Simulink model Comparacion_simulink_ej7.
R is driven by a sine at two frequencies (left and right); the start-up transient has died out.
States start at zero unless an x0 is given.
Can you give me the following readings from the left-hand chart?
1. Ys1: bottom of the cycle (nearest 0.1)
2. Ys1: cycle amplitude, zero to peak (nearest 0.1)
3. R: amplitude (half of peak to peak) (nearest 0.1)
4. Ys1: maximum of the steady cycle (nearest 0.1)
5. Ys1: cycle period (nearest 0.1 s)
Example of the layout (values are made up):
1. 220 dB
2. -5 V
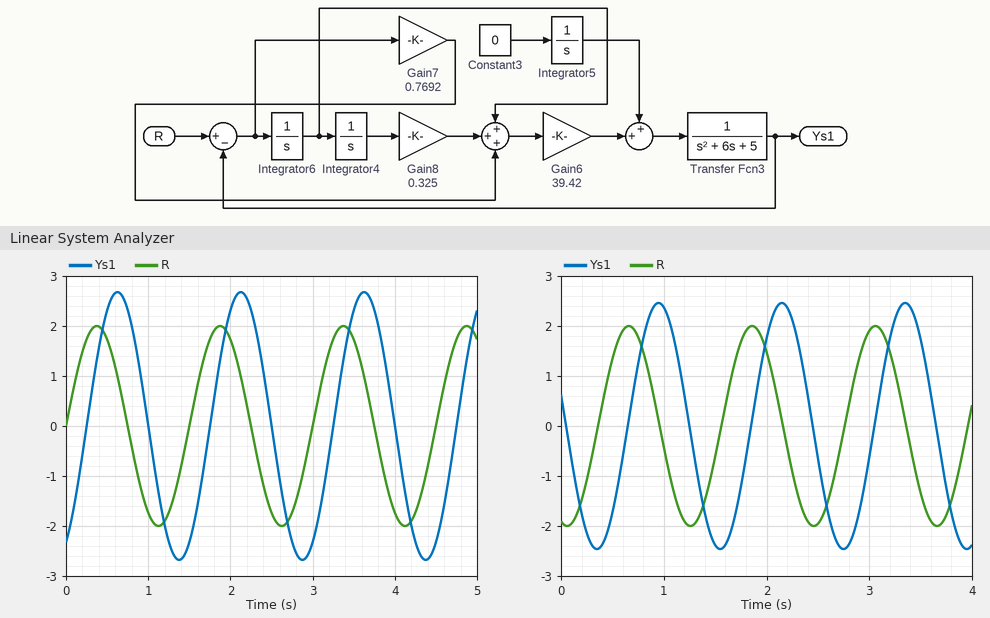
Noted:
1. -2.7
2. 2.7
3. 2.0
4. 2.7
5. 1.5 s
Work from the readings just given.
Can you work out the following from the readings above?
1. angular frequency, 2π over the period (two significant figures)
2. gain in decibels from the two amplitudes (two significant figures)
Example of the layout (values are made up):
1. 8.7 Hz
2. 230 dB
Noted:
1. 4.2 rad/s
2. 2.6 dB
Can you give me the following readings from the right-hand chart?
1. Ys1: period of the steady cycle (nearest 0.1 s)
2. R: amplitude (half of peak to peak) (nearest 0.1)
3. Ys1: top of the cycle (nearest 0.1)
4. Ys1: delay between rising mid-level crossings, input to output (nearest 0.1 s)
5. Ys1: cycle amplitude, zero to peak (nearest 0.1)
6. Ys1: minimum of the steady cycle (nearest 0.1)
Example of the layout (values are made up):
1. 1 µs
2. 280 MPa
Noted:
1. 1.2 s
2. 2.0
3. 2.5
4. 0.3 s
5. 2.5
6. -2.5
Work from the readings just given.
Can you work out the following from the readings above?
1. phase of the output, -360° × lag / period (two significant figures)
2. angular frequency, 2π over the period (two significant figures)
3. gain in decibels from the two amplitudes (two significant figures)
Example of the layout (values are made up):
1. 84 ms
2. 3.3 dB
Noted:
1. -90°
2. 5.2 rad/s
3. 1.9 dB
